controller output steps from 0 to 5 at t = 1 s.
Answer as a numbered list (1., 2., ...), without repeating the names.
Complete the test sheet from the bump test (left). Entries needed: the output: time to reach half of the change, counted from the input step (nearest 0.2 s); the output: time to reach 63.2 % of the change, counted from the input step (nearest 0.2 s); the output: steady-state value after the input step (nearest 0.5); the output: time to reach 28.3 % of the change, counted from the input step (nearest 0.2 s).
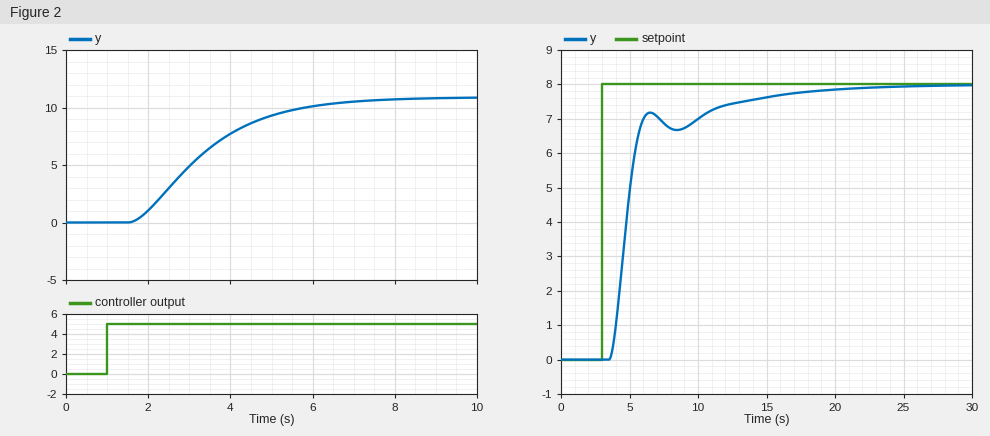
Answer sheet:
1. 2.2 s
2. 2.6 s
3. 11.0
4. 1.6 s
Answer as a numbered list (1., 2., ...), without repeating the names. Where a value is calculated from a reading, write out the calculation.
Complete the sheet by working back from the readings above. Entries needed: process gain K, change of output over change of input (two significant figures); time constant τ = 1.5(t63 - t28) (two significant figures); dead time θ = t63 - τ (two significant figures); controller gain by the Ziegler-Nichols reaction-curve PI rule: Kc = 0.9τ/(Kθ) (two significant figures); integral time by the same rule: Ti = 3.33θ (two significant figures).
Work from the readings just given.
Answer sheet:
1. (11 - 0) / 5 = 2.2
2. 1.5 × (2.6 - 1.6) = 1.5 s
3. 2.6 - 1.5 = 1.1 s
4. 0.9 × 1.5 / (2.2 × 1.1) = 0.56
5. 3.33 × 1.1 = 3.7 s
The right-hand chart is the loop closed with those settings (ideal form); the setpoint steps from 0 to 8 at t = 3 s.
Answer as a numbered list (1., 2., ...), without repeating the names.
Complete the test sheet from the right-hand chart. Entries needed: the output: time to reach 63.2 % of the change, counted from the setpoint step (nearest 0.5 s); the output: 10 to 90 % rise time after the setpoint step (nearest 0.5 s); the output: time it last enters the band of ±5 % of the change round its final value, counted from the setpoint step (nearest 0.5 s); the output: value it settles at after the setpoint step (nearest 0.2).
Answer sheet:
1. 2.0 s
2. 7.0 s
3. 11.5 s
4. 8.0
